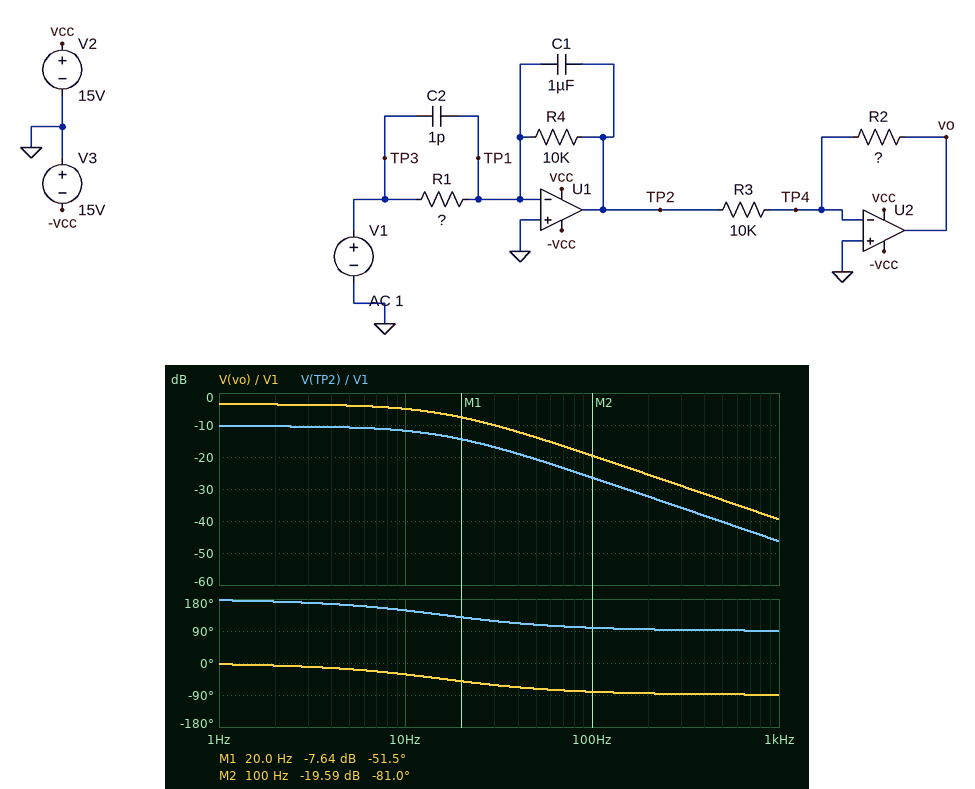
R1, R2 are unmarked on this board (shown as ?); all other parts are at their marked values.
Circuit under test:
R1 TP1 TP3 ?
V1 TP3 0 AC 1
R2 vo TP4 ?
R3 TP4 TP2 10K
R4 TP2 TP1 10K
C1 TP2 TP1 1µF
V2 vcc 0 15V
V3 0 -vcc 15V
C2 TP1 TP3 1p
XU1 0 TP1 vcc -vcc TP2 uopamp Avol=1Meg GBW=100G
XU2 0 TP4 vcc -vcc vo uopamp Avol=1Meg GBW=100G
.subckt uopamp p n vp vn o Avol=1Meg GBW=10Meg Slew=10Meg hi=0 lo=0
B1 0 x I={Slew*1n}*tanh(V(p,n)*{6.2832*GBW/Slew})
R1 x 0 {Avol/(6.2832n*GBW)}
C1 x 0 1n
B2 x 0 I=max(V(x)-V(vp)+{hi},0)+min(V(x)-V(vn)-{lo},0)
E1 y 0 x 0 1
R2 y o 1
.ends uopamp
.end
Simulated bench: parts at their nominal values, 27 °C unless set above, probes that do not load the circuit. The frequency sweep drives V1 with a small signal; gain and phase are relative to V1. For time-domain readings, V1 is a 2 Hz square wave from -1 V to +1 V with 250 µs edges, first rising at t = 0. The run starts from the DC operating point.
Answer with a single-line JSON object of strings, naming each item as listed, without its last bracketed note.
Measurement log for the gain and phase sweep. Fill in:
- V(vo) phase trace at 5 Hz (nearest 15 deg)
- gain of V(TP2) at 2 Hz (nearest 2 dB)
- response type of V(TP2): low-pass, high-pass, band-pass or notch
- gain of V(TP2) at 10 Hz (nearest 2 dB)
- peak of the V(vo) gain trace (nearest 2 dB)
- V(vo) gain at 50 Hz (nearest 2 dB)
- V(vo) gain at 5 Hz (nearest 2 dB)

{"V(vo) phase trace at 5 Hz": "-15 deg", "gain of V(TP2) at 2 Hz": "-10 dB", "response type of V(TP2): low-pass, high-pass, band-pass or notch": "low-pass", "gain of V(TP2) at 10 Hz": "-12 dB", "peak of the V(vo) gain trace": "-4 dB", "V(vo) gain at 50 Hz": "-14 dB", "V(vo) gain at 5 Hz": "-4 dB"}
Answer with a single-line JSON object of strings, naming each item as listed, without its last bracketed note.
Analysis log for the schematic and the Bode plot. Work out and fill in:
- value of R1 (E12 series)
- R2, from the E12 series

{"value of R1": "33 kΩ", "R2, from the E12 series": "22 kΩ"}
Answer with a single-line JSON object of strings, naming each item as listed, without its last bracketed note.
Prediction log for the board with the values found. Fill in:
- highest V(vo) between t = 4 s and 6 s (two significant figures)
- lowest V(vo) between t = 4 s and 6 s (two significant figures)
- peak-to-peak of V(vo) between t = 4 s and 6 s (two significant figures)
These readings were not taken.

{"highest V(vo) between t = 4 s and 6 s": "670 mV", "lowest V(vo) between t = 4 s and 6 s": "-670 mV", "peak-to-peak of V(vo) between t = 4 s and 6 s": "1.3 V"}
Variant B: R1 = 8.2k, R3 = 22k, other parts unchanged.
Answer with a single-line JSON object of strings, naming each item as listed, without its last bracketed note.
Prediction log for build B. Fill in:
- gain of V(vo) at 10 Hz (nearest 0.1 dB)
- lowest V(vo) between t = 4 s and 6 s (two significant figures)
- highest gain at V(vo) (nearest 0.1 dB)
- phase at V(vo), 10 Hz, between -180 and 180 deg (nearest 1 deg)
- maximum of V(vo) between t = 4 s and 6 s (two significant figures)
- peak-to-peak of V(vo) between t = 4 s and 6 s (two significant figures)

{"gain of V(vo) at 10 Hz": "0.3 dB", "lowest V(vo) between t = 4 s and 6 s": "-1.2 V", "highest gain at V(vo)": "1.7 dB", "phase at V(vo), 10 Hz, between -180 and 180 deg": "-32 deg", "maximum of V(vo) between t = 4 s and 6 s": "1.2 V", "peak-to-peak of V(vo) between t = 4 s and 6 s": "2.4 V"}
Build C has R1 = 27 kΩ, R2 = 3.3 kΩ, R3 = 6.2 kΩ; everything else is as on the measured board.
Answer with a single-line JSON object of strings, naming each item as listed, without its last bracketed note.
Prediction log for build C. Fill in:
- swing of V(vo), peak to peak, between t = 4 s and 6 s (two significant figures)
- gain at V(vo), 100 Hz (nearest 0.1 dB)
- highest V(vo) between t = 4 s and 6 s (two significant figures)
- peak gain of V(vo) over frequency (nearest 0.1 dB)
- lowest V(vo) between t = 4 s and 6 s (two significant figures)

{"swing of V(vo), peak to peak, between t = 4 s and 6 s": "390 mV", "gain at V(vo), 100 Hz": "-30.2 dB", "highest V(vo) between t = 4 s and 6 s": "200 mV", "peak gain of V(vo) over frequency": "-14.1 dB", "lowest V(vo) between t = 4 s and 6 s": "-200 mV"}
